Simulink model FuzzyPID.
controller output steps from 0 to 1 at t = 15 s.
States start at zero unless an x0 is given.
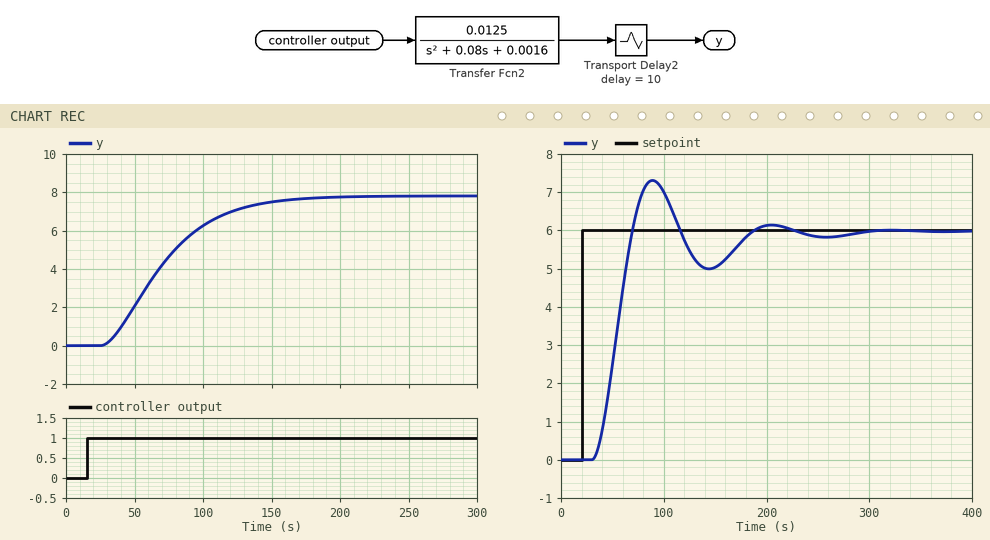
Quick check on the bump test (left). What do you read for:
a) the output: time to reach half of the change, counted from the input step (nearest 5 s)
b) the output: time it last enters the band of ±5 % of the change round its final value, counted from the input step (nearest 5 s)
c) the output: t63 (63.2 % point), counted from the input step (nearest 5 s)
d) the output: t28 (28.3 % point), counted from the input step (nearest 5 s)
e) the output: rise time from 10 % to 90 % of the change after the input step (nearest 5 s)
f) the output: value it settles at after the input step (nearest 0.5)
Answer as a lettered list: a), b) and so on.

a) 50 s
b) 130 s
c) 65 s
d) 35 s
e) 85 s
f) 8.0
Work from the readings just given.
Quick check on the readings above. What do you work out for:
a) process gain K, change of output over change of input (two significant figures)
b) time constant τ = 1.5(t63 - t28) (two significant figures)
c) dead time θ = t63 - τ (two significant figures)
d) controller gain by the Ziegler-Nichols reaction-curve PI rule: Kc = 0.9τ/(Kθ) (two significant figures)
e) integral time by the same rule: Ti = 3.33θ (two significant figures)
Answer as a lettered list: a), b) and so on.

a) 8.0
b) 45 s
c) 20 s
d) 0.25
e) 67 s
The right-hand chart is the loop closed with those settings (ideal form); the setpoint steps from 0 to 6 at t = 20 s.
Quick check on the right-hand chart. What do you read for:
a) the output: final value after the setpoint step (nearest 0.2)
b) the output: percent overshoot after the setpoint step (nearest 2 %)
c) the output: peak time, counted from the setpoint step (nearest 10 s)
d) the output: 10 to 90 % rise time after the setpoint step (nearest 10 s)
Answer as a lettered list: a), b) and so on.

a) 6.0
b) 22 %
c) 70 s
d) 30 s
